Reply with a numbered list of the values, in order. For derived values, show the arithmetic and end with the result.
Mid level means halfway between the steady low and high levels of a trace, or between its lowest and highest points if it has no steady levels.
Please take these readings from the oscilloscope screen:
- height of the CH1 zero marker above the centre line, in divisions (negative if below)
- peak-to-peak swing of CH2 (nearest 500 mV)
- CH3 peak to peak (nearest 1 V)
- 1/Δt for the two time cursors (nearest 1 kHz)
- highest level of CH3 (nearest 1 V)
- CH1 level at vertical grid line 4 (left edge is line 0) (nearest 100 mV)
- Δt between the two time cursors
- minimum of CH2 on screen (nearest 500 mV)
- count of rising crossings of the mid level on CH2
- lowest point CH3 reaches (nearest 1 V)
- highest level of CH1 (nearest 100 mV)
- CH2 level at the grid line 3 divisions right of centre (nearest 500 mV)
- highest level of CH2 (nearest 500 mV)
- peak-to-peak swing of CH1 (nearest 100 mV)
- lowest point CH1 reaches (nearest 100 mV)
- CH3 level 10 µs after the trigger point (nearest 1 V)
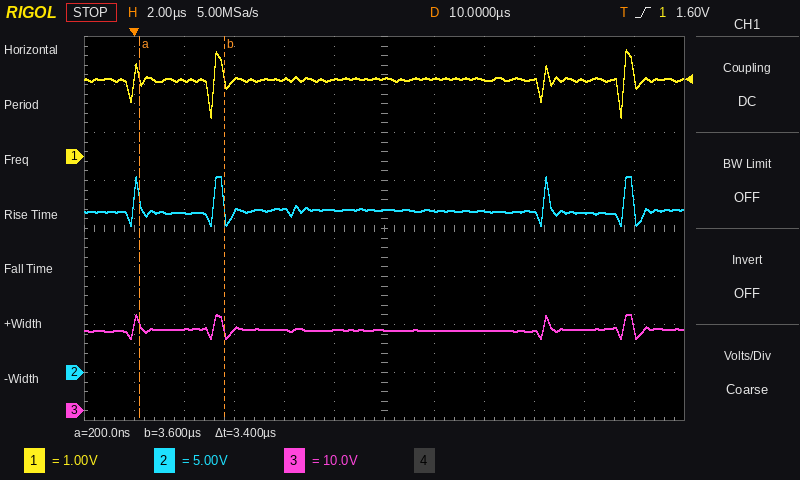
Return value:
1. +1.5 div
2. 20.5 V − (15.5 V) = 5.0 V
3. 20 V − (15 V) = 5 V
4. 1 / 3.4 µs ≈ 294 kHz
5. 20 V
6. 1.6 V
7. 3.4 µs
8. 15.5 V
9. 4
10. 15 V
11. 2.2 V
12. 16.5 V
13. 20.5 V
14. 2.2 V − (800 mV) = 1.4 V
15. 800 mV
16. 17 V
